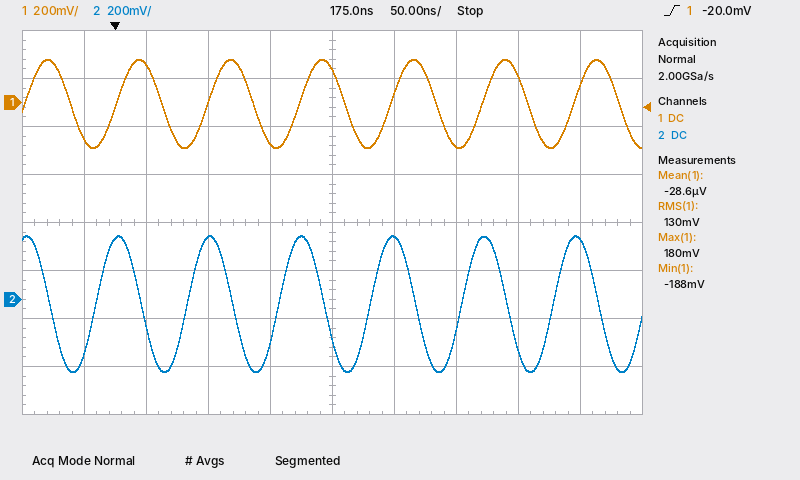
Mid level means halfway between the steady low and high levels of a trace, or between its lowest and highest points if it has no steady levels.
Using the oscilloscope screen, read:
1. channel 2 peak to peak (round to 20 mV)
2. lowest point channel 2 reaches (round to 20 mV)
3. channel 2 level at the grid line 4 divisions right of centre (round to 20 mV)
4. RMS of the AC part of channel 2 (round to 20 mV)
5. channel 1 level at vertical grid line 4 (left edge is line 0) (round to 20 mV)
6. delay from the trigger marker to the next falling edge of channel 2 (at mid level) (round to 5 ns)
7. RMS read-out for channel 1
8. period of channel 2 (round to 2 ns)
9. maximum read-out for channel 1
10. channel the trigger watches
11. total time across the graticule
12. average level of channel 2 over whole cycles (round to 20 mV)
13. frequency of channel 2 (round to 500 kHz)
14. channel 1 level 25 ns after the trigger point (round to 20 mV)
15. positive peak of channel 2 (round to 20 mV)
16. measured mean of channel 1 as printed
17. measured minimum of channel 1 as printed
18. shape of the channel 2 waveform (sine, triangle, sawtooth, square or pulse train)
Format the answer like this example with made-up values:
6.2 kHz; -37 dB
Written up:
560 mV; -300 mV; 240 mV; 200 mV; -160 mV; 20 ns; 130 mV; 74 ns; 180 mV; channel 1; 500 ns; -20 mV; 13.5 MHz; 160 mV; 260 mV; -28.6 µV; -188 mV; sine
